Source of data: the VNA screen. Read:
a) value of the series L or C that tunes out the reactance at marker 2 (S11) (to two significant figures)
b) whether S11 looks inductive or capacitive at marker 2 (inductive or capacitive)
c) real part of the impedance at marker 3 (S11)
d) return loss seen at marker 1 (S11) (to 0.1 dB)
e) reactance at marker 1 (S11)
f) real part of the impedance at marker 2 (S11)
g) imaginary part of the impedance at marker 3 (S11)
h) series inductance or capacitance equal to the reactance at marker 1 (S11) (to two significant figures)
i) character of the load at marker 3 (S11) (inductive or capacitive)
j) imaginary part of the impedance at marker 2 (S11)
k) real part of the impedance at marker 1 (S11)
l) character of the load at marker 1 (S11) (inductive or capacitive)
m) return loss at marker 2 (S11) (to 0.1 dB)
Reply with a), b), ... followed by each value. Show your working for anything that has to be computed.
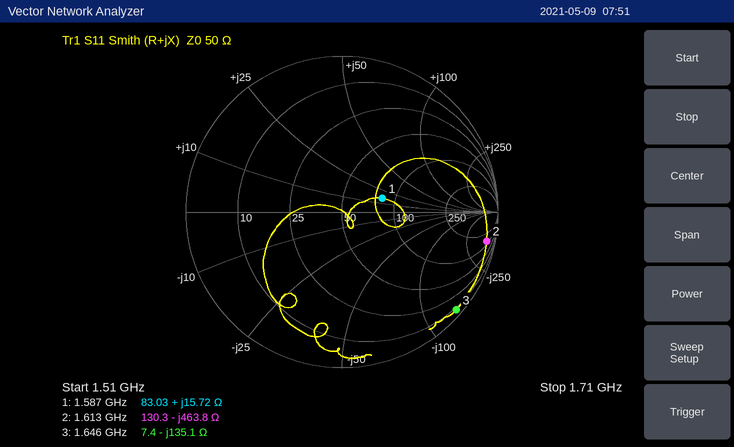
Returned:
a) L = 463.8 Ω/(2π × 1.613 GHz) ≈ 46 nH
b) capacitive
c) 7.4 Ω
d) 11.3 dB
e) +15.72 Ω
f) 130.3 Ω
g) -135.1 Ω
h) L = 15.72 Ω/(2π × 1.587 GHz) ≈ 1.6 nH
i) capacitive
j) -463.8 Ω
k) 83.03 Ω
l) inductive
m) 0.5 dB
